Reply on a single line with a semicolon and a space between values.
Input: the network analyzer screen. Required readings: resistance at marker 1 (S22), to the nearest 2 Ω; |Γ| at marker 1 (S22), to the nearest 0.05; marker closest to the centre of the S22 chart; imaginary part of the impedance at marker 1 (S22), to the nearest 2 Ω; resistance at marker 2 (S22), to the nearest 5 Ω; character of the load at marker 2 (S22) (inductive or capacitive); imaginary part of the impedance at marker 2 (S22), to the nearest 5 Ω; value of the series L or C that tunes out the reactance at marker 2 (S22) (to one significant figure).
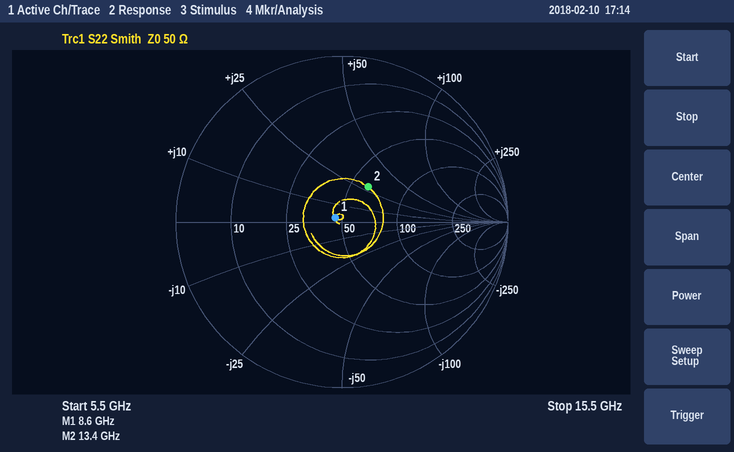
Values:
46 Ω; 0.05; marker 1; +2 Ω; 60 Ω; inductive; +30 Ω; 400 fF
